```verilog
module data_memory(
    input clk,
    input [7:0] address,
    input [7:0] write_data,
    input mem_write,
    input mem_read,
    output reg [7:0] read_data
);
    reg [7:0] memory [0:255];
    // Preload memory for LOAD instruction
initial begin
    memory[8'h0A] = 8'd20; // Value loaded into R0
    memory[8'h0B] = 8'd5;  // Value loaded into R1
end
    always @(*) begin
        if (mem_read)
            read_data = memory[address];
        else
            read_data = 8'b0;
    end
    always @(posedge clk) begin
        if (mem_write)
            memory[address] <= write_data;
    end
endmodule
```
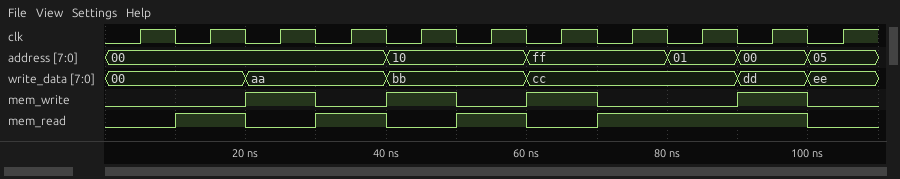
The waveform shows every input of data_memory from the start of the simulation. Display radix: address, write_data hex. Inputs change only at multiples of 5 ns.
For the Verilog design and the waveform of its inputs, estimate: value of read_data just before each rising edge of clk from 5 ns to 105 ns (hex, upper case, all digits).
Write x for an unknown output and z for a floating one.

00, x, 00, AA, 00, BB, 00, CC, x, AA, 00
